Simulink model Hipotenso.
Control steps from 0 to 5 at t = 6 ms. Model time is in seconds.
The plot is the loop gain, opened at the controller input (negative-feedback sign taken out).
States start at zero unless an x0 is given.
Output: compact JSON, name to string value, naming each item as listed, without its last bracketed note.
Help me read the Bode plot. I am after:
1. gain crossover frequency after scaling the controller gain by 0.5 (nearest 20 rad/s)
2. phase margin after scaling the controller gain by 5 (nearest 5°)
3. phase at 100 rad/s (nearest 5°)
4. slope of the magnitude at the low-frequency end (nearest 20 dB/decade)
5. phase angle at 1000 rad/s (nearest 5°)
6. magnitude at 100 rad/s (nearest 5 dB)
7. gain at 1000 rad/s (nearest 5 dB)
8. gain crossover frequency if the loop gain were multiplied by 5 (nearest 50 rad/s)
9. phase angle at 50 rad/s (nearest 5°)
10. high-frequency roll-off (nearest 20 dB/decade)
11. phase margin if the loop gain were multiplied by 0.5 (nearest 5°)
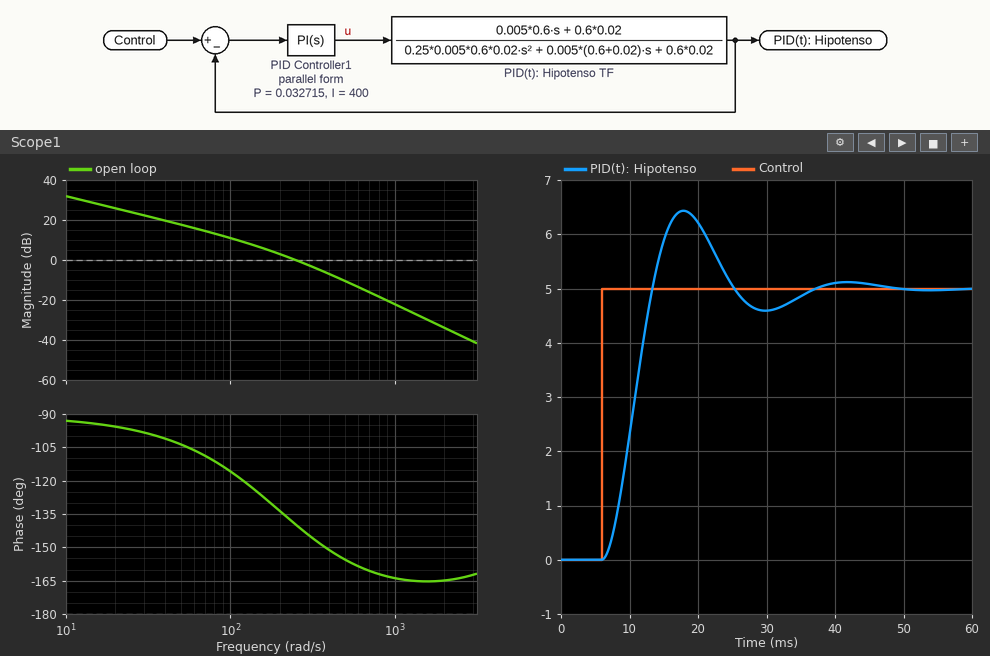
{"gain crossover frequency after scaling the controller gain by 0.5": "160 rad/s", "phase margin after scaling the controller gain by 5": "20°", "phase at 100 rad/s": "-115°", "slope of the magnitude at the low-frequency end": "-20 dB/decade", "phase angle at 1000 rad/s": "-165°", "magnitude at 100 rad/s": "10 dB", "gain at 1000 rad/s": "-20 dB", "gain crossover frequency if the loop gain were multiplied by 5": "600 rad/s", "phase angle at 50 rad/s": "-105°", "high-frequency roll-off": "-40 dB/decade", "phase margin if the loop gain were multiplied by 0.5": "55°"}
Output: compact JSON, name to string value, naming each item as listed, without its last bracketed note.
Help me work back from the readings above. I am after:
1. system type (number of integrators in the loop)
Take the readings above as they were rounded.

{"system type": "1"}
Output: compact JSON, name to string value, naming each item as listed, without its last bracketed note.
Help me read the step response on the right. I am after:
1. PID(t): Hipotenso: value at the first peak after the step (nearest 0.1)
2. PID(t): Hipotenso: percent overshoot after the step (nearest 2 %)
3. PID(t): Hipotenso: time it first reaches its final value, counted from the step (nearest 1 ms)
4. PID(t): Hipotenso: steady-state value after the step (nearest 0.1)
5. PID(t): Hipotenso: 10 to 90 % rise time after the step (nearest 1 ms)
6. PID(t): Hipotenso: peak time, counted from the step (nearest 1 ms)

{"PID(t): Hipotenso: value at the first peak after the step": "6.4", "PID(t): Hipotenso: percent overshoot after the step": "28 %", "PID(t): Hipotenso: time it first reaches its final value, counted from the step": "7 ms", "PID(t): Hipotenso: steady-state value after the step": "5.0", "PID(t): Hipotenso: 10 to 90 % rise time after the step": "5 ms", "PID(t): Hipotenso: peak time, counted from the step": "12 ms"}
